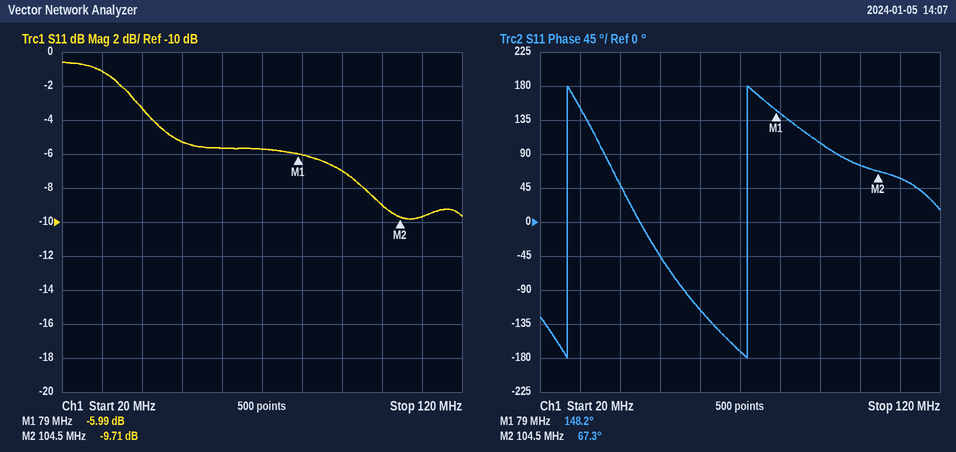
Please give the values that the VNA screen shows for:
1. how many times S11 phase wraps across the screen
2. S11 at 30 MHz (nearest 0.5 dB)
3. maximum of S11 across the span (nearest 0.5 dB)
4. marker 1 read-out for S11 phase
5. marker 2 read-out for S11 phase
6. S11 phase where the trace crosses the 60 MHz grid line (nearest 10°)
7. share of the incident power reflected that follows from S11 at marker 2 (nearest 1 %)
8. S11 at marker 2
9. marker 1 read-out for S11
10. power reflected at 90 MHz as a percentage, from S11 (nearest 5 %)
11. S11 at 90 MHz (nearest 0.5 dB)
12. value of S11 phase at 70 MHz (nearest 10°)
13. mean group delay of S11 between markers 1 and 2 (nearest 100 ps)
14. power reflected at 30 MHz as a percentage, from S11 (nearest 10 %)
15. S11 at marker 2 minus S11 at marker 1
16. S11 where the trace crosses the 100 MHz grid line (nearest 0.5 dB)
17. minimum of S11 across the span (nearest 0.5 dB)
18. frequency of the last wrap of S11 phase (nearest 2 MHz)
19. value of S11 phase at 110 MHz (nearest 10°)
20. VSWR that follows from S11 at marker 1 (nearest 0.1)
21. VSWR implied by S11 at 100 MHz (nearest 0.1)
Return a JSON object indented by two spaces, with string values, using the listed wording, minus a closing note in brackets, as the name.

{
  "how many times S11 phase wraps across the screen": "2",
  "S11 at 30 MHz": "-1.0 dB",
  "maximum of S11 across the span": "-0.5 dB",
  "marker 1 read-out for S11 phase": "148.2°",
  "marker 2 read-out for S11 phase": "67.3°",
  "S11 phase where the trace crosses the 60 MHz grid line": "-120°",
  "share of the incident power reflected that follows from S11 at marker 2": "11 %",
  "S11 at marker 2": "-9.71 dB",
  "marker 1 read-out for S11": "-5.99 dB",
  "power reflected at 90 MHz as a percentage, from S11": "20 %",
  "S11 at 90 MHz": "-7.0 dB",
  "value of S11 phase at 70 MHz": "-170°",
  "mean group delay of S11 between markers 1 and 2": "8.8 ns",
  "power reflected at 30 MHz as a percentage, from S11": "80 %",
  "S11 at marker 2 minus S11 at marker 1": "-3.72 dB",
  "S11 where the trace crosses the 100 MHz grid line": "-9.0 dB",
  "minimum of S11 across the span": "-10.0 dB",
  "frequency of the last wrap of S11 phase": "72 MHz",
  "value of S11 phase at 110 MHz": "60°",
  "VSWR that follows from S11 at marker 1": "3.0",
  "VSWR implied by S11 at 100 MHz": "2.1"
}
